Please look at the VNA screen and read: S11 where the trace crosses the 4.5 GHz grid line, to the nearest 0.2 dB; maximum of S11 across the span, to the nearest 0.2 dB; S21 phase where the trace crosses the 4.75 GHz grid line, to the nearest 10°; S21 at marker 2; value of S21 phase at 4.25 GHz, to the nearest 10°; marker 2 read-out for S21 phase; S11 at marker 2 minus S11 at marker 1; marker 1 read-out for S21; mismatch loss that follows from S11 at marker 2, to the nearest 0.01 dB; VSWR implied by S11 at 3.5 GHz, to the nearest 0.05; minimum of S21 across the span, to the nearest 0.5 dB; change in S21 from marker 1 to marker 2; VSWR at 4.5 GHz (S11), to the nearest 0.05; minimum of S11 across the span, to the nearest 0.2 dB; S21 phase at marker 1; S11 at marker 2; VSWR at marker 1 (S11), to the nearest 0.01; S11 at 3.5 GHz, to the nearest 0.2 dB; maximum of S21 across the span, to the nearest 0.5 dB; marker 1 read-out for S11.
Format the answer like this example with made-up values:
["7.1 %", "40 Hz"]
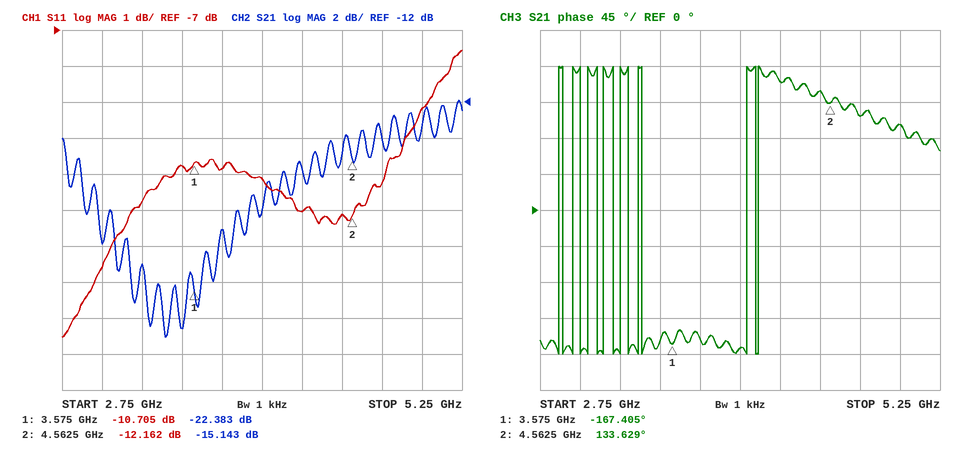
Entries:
["-12.2 dB", "-7.6 dB", "120°", "-15.143 dB", "160°", "133.629°", "-1.457 dB", "-22.383 dB", "0.27 dB", "1.80", "-25.0 dB", "7.240 dB", "1.65", "-15.6 dB", "-167.405°", "-12.162 dB", "1.82", "-10.8 dB", "-12.0 dB", "-10.705 dB"]
